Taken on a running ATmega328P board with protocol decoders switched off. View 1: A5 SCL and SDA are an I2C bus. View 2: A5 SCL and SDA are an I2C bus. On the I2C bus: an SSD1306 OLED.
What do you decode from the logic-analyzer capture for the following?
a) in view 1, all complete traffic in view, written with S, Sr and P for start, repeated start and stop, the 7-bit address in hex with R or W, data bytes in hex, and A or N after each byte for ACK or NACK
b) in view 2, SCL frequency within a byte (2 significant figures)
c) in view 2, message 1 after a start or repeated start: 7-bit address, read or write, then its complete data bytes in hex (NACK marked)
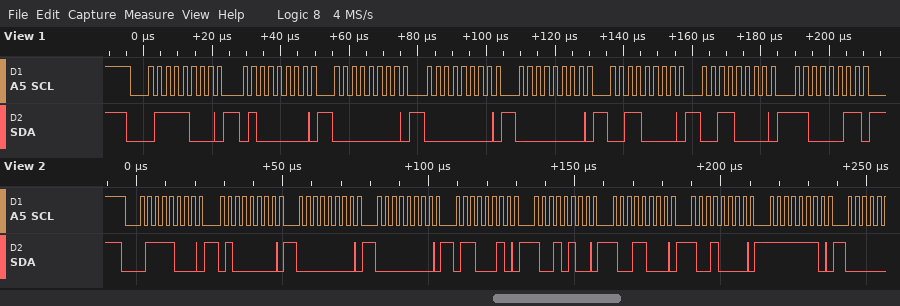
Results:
S 3CW A 40 A 00 A 00 A 00 A 30 A 30 A C3 A
400 kHz
0x3C write: 40 00 00 62 94 98 90 FE
